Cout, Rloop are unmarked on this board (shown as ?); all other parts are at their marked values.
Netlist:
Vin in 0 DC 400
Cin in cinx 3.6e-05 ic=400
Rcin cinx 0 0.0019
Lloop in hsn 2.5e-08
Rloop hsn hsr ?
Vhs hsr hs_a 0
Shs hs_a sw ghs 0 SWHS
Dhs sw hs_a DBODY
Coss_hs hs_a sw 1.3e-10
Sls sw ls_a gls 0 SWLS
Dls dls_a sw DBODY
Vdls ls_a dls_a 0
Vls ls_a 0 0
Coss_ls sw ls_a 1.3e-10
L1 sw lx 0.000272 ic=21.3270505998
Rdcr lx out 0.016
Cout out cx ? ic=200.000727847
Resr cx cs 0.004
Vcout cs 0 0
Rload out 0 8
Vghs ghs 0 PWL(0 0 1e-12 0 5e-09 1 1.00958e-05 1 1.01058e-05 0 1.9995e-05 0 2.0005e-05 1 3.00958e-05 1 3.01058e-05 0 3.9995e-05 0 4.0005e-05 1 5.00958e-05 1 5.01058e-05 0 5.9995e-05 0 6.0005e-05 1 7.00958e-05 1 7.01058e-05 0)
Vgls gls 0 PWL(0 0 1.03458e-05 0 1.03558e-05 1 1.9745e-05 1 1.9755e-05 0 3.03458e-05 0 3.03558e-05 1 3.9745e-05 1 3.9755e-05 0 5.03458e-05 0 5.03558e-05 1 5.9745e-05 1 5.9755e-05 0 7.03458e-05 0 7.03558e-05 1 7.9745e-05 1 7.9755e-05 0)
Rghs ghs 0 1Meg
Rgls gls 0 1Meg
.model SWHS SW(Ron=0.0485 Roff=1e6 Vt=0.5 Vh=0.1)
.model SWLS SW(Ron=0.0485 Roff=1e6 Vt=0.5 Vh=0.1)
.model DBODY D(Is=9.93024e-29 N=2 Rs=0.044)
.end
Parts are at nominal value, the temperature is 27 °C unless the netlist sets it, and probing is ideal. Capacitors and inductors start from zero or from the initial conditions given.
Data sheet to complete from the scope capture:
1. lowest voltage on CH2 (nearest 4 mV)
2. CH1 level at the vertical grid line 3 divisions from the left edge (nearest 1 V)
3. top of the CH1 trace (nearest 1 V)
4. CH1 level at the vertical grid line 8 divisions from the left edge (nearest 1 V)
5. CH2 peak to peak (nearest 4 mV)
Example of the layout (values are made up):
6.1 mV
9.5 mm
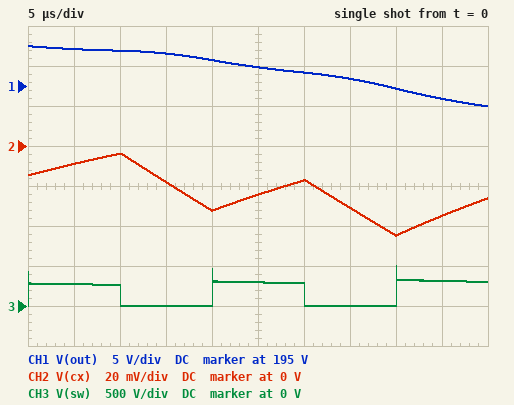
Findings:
-44 mV
199 V
200 V
195 V
40 mV
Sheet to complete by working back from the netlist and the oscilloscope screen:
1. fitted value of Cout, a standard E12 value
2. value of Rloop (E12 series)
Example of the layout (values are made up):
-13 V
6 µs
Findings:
39 µF
5.6 Ω
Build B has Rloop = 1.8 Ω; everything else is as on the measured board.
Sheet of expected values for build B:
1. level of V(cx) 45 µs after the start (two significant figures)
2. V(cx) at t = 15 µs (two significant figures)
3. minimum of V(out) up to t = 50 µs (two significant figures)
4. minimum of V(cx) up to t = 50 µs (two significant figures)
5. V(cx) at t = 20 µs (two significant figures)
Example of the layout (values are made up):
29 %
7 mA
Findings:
-13 mV
-6.1 mV
200 V
-26 mV
-21 mV
